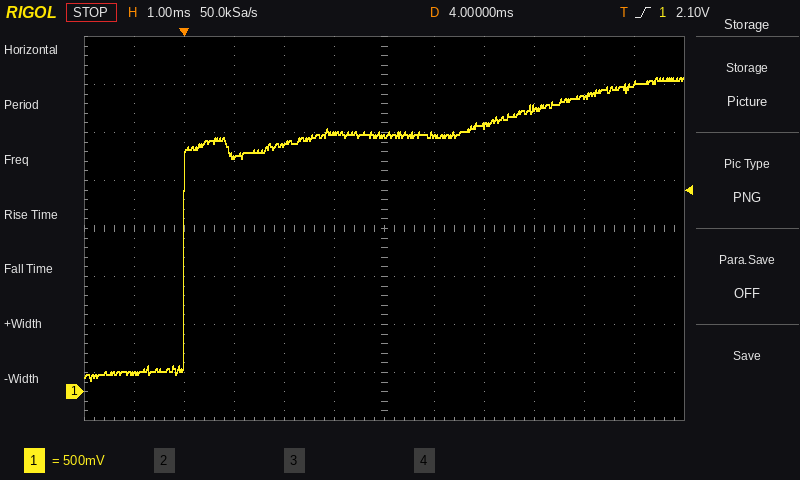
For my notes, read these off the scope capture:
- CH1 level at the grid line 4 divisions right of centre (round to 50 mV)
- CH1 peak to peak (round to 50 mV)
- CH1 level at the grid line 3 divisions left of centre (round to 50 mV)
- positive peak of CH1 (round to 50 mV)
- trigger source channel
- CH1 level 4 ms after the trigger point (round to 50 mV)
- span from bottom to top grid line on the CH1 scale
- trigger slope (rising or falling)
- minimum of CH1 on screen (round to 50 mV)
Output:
3.05 V
3.15 V
2.45 V
3.25 V
CH1
2.65 V
4 V
rising
100 mV
